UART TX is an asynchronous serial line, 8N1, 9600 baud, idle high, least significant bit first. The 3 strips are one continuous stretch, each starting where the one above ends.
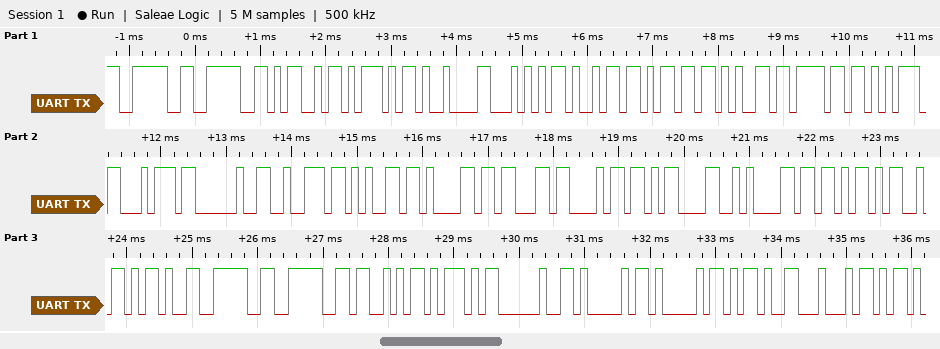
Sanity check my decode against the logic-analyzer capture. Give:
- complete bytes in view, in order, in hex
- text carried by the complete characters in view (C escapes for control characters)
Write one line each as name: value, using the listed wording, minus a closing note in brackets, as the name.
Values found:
complete bytes in view, in order, in hex: 3E 3E 4D 5D 09 54 69 6D 65 6F 75 74 20 72 65 61 63 68 0D 0A 5B 4D 2D 3E 3E 53 5D 20 41 41 2D 44
text carried by the complete characters in view: ">>M]\tTimeout reach\r\n[M->>S] AA-D"
